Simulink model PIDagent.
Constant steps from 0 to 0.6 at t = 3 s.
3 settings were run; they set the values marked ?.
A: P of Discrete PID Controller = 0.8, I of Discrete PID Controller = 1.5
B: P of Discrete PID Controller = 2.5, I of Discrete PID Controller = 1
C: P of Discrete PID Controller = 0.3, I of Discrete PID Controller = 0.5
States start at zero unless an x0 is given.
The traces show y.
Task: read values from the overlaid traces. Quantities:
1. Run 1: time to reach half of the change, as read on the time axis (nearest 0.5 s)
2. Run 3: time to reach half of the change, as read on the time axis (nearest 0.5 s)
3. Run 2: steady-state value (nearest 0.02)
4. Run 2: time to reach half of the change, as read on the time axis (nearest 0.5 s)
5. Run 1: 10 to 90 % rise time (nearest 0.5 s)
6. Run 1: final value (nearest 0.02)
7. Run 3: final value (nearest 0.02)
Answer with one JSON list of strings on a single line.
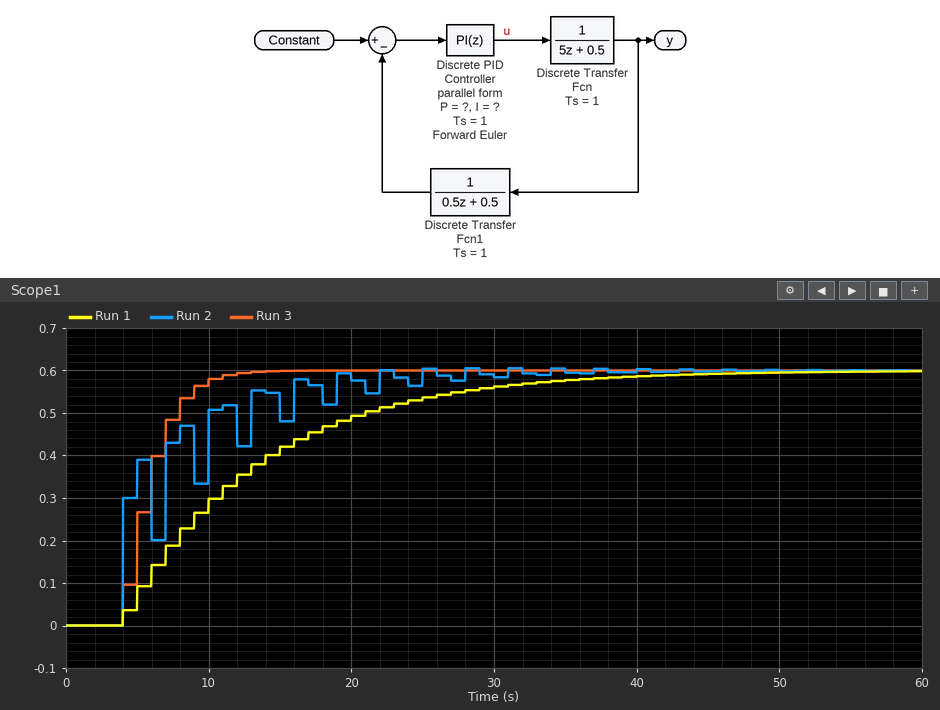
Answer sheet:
["11.0 s", "6.0 s", "0.60", "5.0 s", "21.0 s", "0.60", "0.60"]
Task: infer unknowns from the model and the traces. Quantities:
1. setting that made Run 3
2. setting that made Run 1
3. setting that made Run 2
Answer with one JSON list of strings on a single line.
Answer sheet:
["A", "C", "B"]
